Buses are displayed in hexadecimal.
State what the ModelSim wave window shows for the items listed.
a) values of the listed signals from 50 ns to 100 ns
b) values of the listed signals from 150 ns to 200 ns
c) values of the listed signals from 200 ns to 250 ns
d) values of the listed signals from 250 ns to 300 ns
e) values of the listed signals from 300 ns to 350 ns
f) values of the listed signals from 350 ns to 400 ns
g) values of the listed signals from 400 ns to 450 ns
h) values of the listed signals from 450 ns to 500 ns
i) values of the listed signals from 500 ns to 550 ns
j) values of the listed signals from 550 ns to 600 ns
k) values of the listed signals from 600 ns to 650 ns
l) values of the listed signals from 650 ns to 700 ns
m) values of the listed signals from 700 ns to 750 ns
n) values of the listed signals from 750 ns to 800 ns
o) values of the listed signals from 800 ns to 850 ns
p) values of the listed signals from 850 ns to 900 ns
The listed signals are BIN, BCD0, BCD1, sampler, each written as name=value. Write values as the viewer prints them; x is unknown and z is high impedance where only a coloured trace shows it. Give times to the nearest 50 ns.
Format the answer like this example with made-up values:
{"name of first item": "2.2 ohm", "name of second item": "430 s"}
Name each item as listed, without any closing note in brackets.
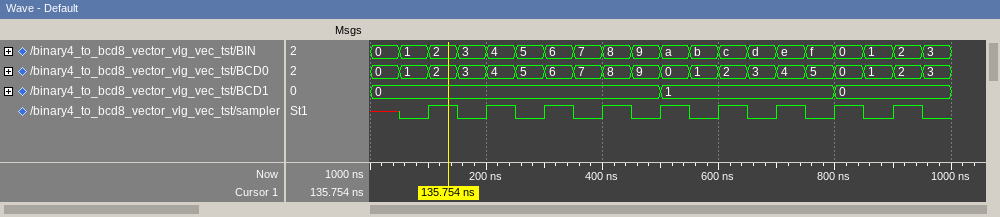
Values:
{"values of the listed signals from 50 ns to 100 ns": "BIN=1, BCD0=1, BCD1=0, sampler=0", "values of the listed signals from 150 ns to 200 ns": "BIN=3, BCD0=3, BCD1=0, sampler=0", "values of the listed signals from 200 ns to 250 ns": "BIN=4, BCD0=4, BCD1=0, sampler=1", "values of the listed signals from 250 ns to 300 ns": "BIN=5, BCD0=5, BCD1=0, sampler=0", "values of the listed signals from 300 ns to 350 ns": "BIN=6, BCD0=6, BCD1=0, sampler=1", "values of the listed signals from 350 ns to 400 ns": "BIN=7, BCD0=7, BCD1=0, sampler=0", "values of the listed signals from 400 ns to 450 ns": "BIN=8, BCD0=8, BCD1=0, sampler=1", "values of the listed signals from 450 ns to 500 ns": "BIN=9, BCD0=9, BCD1=0, sampler=0", "values of the listed signals from 500 ns to 550 ns": "BIN=a, BCD0=0, BCD1=1, sampler=1", "values of the listed signals from 550 ns to 600 ns": "BIN=b, BCD0=1, BCD1=1, sampler=0", "values of the listed signals from 600 ns to 650 ns": "BIN=c, BCD0=2, BCD1=1, sampler=1", "values of the listed signals from 650 ns to 700 ns": "BIN=d, BCD0=3, BCD1=1, sampler=0", "values of the listed signals from 700 ns to 750 ns": "BIN=e, BCD0=4, BCD1=1, sampler=1", "values of the listed signals from 750 ns to 800 ns": "BIN=f, BCD0=5, BCD1=1, sampler=0", "values of the listed signals from 800 ns to 850 ns": "BIN=0, BCD0=0, BCD1=0, sampler=1", "values of the listed signals from 850 ns to 900 ns": "BIN=1, BCD0=1, BCD1=0, sampler=0"}
